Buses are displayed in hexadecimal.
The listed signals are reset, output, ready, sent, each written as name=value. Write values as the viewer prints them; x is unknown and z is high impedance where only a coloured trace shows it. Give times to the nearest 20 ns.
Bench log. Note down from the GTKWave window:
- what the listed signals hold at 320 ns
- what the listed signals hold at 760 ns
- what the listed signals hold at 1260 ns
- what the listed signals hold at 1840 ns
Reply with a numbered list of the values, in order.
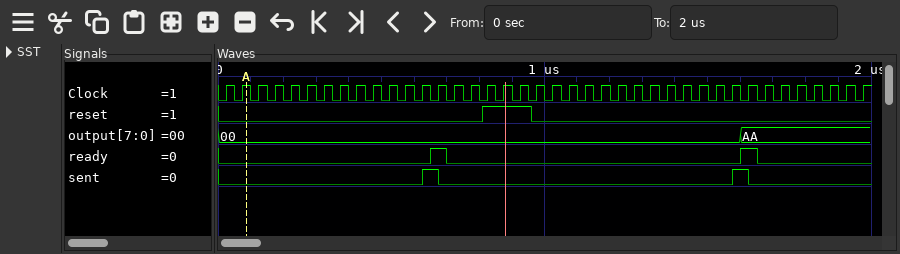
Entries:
1. reset=0, output=00, ready=0, sent=0
2. reset=0, output=00, ready=0, sent=0
3. reset=0, output=00, ready=0, sent=0
4. reset=0, output=AA, ready=0, sent=0
